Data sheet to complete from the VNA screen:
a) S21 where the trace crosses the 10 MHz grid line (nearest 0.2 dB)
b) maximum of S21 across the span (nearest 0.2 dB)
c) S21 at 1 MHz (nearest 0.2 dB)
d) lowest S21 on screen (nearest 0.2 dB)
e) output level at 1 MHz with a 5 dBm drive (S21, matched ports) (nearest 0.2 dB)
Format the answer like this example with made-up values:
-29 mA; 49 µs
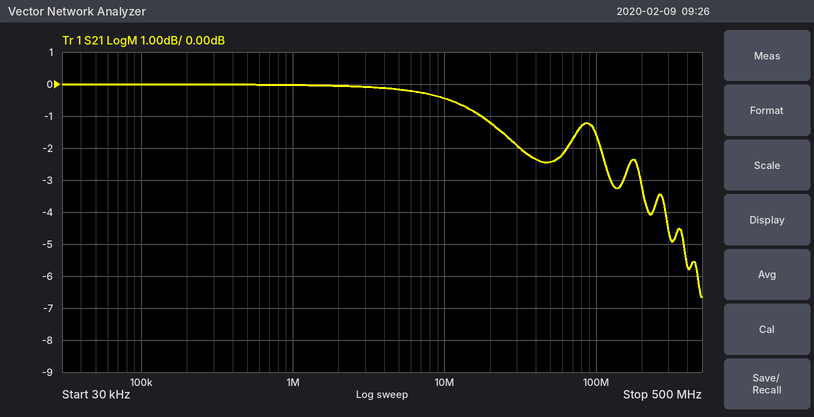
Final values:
-0.4 dB; 0.0 dB; 0.0 dB; -6.6 dB; 5.0 dBm
